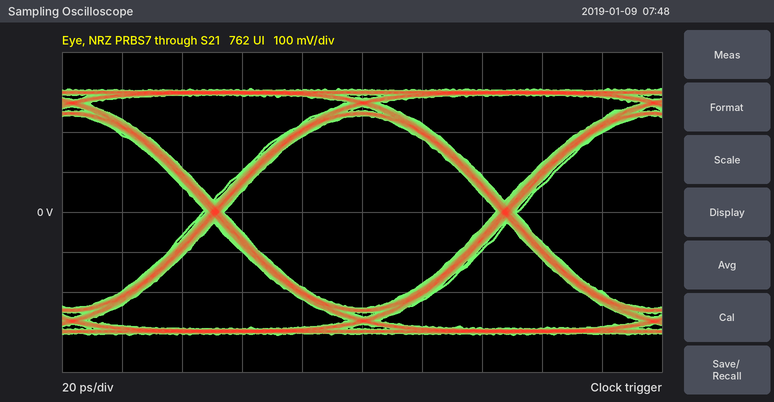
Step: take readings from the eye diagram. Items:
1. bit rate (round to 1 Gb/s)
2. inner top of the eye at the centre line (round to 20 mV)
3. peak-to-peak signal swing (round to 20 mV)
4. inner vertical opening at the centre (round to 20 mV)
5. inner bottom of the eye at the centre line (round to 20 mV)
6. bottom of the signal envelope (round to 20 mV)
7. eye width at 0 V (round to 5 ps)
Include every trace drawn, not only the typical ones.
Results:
10 Gb/s
240 mV
620 mV
480 mV
-240 mV
-300 mV
90 ps
